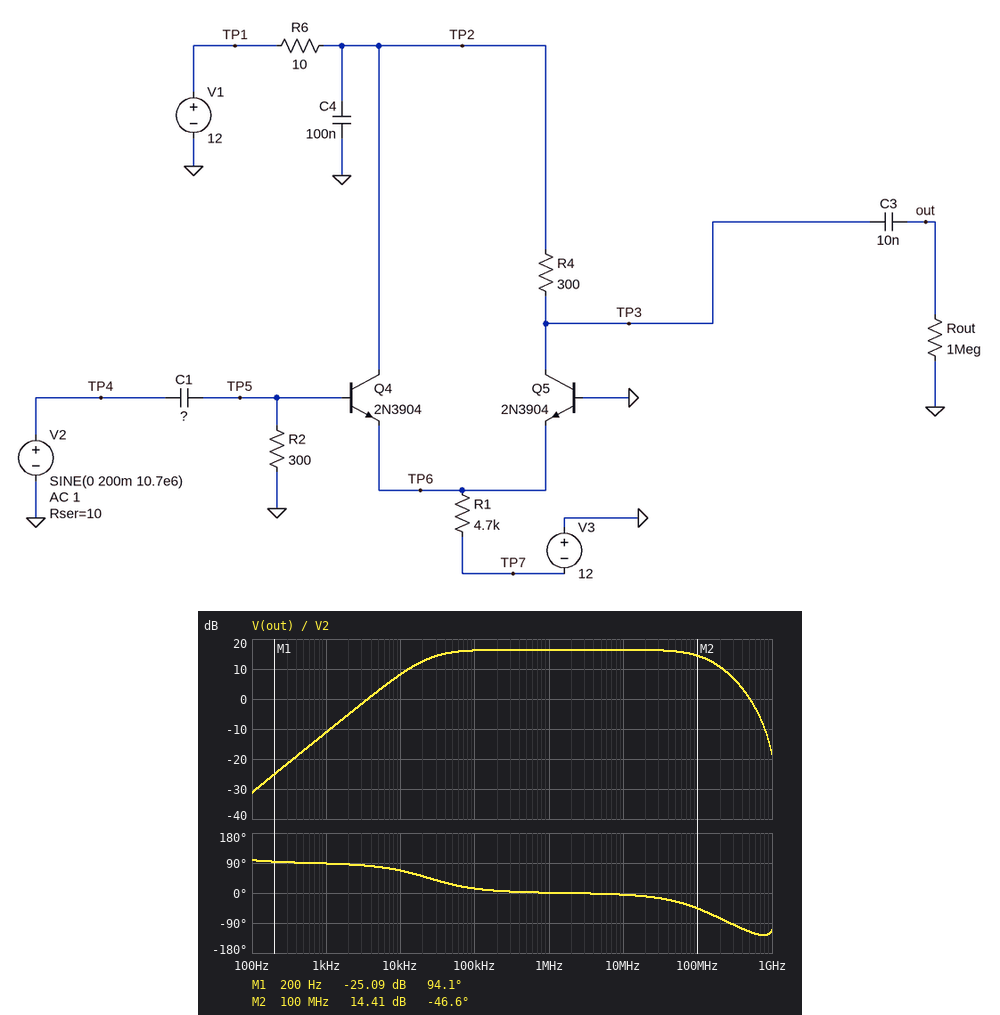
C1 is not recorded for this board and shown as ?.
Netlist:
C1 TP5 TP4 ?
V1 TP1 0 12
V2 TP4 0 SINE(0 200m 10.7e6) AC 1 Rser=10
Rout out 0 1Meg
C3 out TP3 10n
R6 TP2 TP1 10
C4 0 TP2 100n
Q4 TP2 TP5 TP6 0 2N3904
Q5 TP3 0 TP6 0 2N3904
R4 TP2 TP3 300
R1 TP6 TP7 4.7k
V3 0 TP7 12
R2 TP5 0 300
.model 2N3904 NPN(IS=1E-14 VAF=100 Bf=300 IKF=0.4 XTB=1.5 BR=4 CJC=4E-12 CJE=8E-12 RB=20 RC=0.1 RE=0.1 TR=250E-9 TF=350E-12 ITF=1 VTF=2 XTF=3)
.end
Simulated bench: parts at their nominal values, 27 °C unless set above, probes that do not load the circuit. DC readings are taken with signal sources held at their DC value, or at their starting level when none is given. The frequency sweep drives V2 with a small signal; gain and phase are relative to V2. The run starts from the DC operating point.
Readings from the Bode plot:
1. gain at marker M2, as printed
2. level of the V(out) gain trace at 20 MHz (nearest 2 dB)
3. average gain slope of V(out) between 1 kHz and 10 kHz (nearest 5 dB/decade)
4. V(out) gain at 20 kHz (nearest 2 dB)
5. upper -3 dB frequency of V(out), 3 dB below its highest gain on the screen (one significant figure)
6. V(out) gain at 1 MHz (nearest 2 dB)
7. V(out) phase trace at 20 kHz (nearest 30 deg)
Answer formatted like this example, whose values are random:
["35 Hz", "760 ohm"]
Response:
["14.41 dB", "16 dB", "20 dB/decade", "12 dB", "100 MHz", "16 dB", "60 deg"]
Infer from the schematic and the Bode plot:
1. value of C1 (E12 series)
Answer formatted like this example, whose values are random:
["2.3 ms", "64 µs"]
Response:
["22 nF"]
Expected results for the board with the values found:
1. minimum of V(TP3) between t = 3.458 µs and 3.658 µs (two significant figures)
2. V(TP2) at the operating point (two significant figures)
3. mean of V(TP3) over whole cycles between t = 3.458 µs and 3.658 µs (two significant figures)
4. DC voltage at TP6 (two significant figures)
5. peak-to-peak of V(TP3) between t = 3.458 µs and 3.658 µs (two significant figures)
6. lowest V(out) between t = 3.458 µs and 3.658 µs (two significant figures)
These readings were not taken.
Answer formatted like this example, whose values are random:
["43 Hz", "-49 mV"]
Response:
["11 V", "12 V", "12 V", "-660 mV", "750 mV", "-380 mV"]
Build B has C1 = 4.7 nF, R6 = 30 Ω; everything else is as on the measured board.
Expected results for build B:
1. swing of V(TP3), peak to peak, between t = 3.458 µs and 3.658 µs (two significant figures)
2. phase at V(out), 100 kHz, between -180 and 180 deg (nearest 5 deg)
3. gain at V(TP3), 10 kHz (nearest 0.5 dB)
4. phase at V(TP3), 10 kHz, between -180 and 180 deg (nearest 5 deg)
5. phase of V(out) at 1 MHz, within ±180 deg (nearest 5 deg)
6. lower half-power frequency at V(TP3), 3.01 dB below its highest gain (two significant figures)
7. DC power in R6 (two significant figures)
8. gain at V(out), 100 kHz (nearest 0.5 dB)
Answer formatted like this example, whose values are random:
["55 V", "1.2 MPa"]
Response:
["750 mV", "50 deg", "-4.5 dB", "85 deg", "5 deg", "110 kHz", "170 µW", "13.0 dB"]
